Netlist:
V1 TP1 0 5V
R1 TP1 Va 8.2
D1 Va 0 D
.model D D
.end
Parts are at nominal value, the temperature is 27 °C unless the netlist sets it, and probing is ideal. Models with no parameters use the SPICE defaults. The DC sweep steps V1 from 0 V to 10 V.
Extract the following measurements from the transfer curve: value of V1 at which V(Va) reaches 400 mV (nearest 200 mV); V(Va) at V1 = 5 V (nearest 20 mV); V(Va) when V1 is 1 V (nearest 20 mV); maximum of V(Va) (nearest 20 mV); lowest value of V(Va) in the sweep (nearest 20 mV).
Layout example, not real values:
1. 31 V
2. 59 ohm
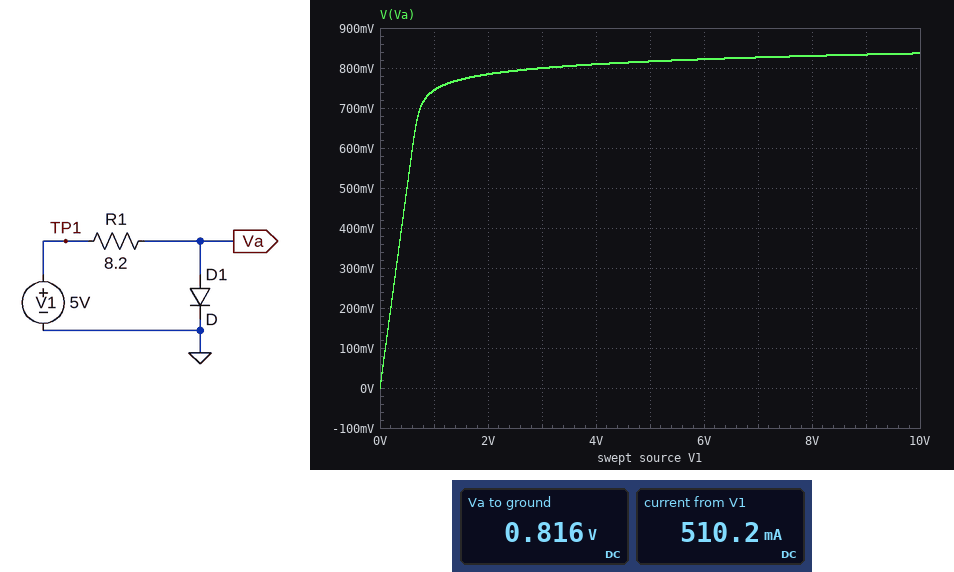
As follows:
1. 400 mV
2. 820 mV
3. 740 mV
4. 840 mV
5. 0 V
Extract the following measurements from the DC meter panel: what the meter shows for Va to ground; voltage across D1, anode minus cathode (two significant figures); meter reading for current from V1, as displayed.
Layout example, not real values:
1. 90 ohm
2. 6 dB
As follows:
1. 0.816 V
2. 820 mV
3. 510.2 mA
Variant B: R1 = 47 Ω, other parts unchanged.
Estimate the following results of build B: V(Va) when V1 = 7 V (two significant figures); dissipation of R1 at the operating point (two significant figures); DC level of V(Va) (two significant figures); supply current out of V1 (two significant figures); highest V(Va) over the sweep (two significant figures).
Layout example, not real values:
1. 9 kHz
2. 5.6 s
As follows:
1. 780 mV
2. 380 mW
3. 770 mV
4. 90 mA
5. 790 mV
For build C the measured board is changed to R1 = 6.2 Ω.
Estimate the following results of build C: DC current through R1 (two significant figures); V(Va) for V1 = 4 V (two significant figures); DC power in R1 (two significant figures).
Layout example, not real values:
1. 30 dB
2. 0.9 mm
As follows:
1. 670 mA
2. 820 mV
3. 2.8 W
